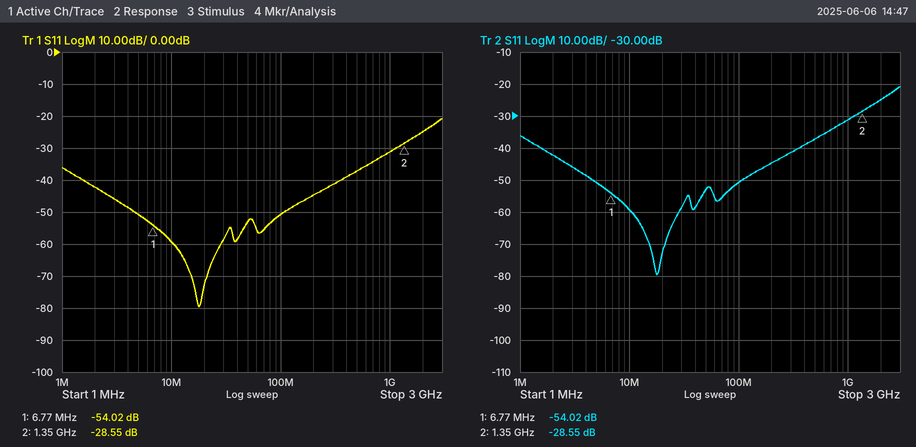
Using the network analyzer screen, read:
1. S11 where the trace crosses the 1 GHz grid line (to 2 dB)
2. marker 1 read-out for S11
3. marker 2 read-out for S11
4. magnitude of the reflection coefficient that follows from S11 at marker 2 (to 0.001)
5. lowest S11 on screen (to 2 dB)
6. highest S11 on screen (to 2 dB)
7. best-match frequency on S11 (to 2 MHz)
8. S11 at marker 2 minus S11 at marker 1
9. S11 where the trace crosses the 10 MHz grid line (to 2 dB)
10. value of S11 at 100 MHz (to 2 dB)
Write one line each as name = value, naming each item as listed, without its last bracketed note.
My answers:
S11 where the trace crosses the 1 GHz grid line = -32 dB
marker 1 read-out for S11 = -54.02 dB
marker 2 read-out for S11 = -28.55 dB
magnitude of the reflection coefficient that follows from S11 at marker 2 = 0.037
lowest S11 on screen = -80 dB
highest S11 on screen = -20 dB
best-match frequency on S11 = 18 MHz
S11 at marker 2 minus S11 at marker 1 = 25.47 dB
S11 where the trace crosses the 10 MHz grid line = -60 dB
value of S11 at 100 MHz = -50 dB
